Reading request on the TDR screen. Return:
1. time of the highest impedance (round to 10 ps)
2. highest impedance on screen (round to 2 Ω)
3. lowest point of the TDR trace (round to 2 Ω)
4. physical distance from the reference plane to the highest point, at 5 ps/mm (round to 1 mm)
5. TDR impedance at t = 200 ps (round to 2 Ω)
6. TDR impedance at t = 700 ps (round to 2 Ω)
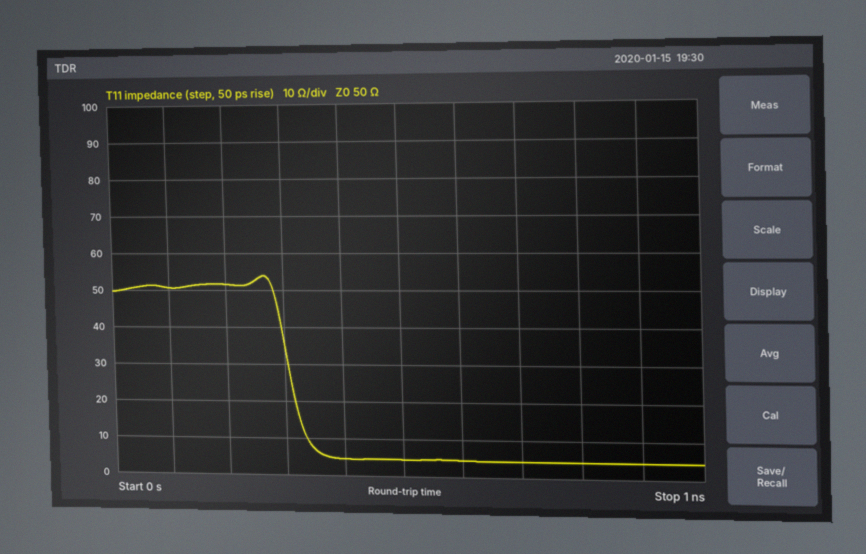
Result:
270 ps
54 Ω
4 Ω
27 mm
52 Ω
4 Ω
